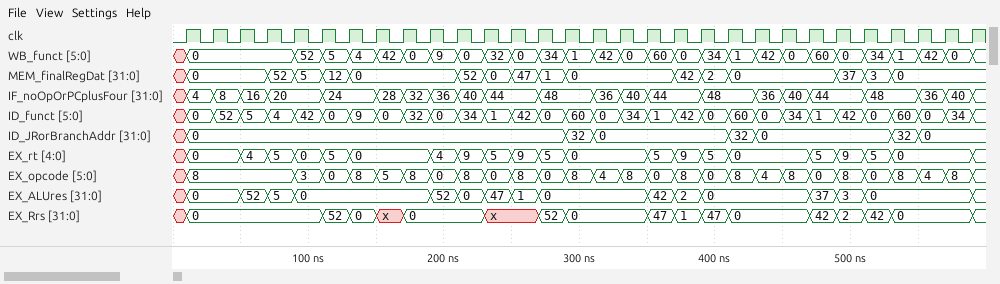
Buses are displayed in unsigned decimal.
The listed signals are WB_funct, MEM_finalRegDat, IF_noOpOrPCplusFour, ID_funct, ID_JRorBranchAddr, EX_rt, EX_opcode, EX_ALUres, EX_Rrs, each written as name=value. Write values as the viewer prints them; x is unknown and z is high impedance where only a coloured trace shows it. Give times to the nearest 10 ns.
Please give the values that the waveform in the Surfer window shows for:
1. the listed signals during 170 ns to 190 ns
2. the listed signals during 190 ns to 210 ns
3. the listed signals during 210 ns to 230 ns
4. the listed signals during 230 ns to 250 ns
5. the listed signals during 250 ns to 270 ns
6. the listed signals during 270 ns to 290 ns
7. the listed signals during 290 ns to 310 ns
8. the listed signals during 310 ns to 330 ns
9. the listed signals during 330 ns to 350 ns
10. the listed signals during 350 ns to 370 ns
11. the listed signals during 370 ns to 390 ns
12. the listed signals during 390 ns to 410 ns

WB_funct=0, MEM_finalRegDat=0, IF_noOpOrPCplusFour=32, ID_funct=32, ID_JRorBranchAddr=0, EX_rt=0, EX_opcode=8, EX_ALUres=0, EX_Rrs=0
WB_funct=9, MEM_finalRegDat=0, IF_noOpOrPCplusFour=36, ID_funct=0, ID_JRorBranchAddr=0, EX_rt=4, EX_opcode=0, EX_ALUres=52, EX_Rrs=0
WB_funct=0, MEM_finalRegDat=52, IF_noOpOrPCplusFour=40, ID_funct=34, ID_JRorBranchAddr=0, EX_rt=9, EX_opcode=8, EX_ALUres=0, EX_Rrs=0
WB_funct=32, MEM_finalRegDat=0, IF_noOpOrPCplusFour=44, ID_funct=1, ID_JRorBranchAddr=0, EX_rt=5, EX_opcode=0, EX_ALUres=47, EX_Rrs=x
WB_funct=0, MEM_finalRegDat=47, IF_noOpOrPCplusFour=44, ID_funct=42, ID_JRorBranchAddr=0, EX_rt=9, EX_opcode=8, EX_ALUres=1, EX_Rrs=x
WB_funct=34, MEM_finalRegDat=1, IF_noOpOrPCplusFour=48, ID_funct=0, ID_JRorBranchAddr=0, EX_rt=5, EX_opcode=0, EX_ALUres=0, EX_Rrs=52
WB_funct=1, MEM_finalRegDat=0, IF_noOpOrPCplusFour=48, ID_funct=60, ID_JRorBranchAddr=32, EX_rt=0, EX_opcode=8, EX_ALUres=0, EX_Rrs=0
WB_funct=42, MEM_finalRegDat=0, IF_noOpOrPCplusFour=36, ID_funct=0, ID_JRorBranchAddr=0, EX_rt=0, EX_opcode=4, EX_ALUres=0, EX_Rrs=0
WB_funct=0, MEM_finalRegDat=0, IF_noOpOrPCplusFour=40, ID_funct=34, ID_JRorBranchAddr=0, EX_rt=0, EX_opcode=8, EX_ALUres=0, EX_Rrs=0
WB_funct=60, MEM_finalRegDat=0, IF_noOpOrPCplusFour=44, ID_funct=1, ID_JRorBranchAddr=0, EX_rt=5, EX_opcode=0, EX_ALUres=42, EX_Rrs=47
WB_funct=0, MEM_finalRegDat=42, IF_noOpOrPCplusFour=44, ID_funct=42, ID_JRorBranchAddr=0, EX_rt=9, EX_opcode=8, EX_ALUres=2, EX_Rrs=1
WB_funct=34, MEM_finalRegDat=2, IF_noOpOrPCplusFour=48, ID_funct=0, ID_JRorBranchAddr=0, EX_rt=5, EX_opcode=0, EX_ALUres=0, EX_Rrs=47
